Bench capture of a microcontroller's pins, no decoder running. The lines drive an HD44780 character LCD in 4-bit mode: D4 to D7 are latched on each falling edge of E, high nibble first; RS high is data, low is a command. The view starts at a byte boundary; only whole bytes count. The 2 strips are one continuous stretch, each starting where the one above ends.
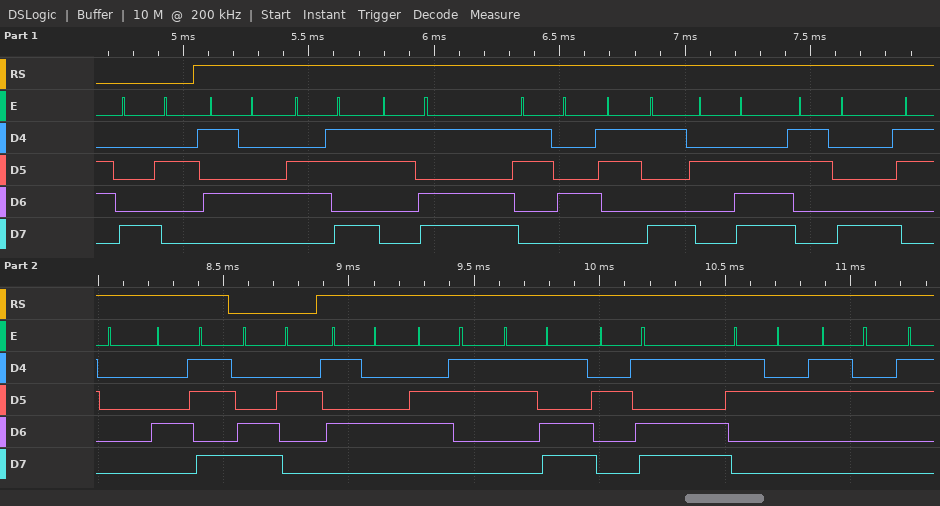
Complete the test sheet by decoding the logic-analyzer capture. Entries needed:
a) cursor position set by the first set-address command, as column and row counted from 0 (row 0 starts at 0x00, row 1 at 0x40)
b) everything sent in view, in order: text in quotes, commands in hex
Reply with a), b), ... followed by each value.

a) column 2, row 0
b) 0x82 "Tk=49.80K" 0xC2 "Tc=-22"
